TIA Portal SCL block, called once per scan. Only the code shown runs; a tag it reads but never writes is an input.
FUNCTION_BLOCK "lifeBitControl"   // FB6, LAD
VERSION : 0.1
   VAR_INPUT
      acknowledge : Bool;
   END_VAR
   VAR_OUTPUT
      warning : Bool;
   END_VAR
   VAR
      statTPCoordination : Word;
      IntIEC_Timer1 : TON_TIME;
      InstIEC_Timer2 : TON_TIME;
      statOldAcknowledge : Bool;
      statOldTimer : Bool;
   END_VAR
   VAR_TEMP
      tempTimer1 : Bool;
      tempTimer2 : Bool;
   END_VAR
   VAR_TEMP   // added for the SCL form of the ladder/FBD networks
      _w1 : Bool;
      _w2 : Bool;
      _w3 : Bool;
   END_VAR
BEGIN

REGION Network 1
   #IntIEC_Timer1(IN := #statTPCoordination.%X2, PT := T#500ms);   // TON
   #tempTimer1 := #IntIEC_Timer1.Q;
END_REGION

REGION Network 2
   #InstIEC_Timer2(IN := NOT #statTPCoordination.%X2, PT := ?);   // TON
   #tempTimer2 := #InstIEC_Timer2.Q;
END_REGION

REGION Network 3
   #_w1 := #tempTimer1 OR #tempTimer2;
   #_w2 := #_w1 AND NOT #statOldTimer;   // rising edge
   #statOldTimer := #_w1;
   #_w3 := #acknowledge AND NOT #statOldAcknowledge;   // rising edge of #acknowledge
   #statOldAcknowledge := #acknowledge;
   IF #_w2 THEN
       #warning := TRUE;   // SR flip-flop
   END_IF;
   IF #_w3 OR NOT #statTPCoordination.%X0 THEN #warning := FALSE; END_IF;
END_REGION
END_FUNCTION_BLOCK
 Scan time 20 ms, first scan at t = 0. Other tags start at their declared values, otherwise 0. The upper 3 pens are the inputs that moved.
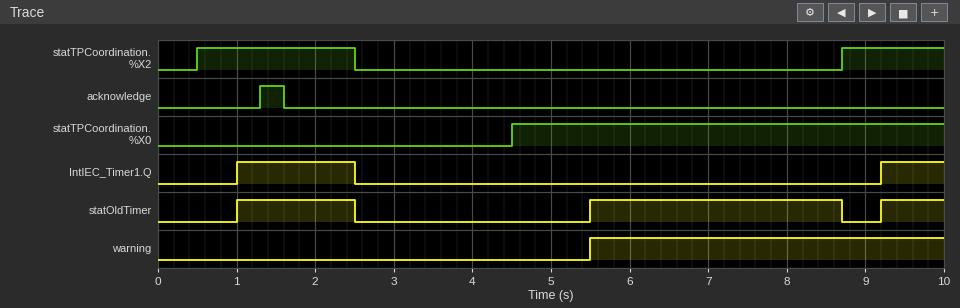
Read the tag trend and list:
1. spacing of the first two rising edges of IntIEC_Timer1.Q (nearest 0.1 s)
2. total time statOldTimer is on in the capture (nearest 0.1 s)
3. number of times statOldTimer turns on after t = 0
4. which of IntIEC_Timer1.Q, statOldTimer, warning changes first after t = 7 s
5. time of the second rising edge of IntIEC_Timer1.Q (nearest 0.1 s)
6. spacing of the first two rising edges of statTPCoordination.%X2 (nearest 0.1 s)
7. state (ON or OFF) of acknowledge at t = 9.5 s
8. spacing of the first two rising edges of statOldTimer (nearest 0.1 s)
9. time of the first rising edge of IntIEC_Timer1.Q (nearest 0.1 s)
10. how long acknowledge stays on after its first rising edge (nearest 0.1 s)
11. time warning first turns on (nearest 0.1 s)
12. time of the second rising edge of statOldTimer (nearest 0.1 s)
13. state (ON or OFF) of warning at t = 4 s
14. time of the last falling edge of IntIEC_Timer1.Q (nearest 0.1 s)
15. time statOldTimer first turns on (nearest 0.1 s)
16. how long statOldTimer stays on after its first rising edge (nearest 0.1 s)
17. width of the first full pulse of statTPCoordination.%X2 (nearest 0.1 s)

8.2 s
5.5 s
3
statOldTimer
9.2 s
8.2 s
OFF
4.5 s
1.0 s
0.3 s
5.5 s
5.5 s
OFF
2.5 s
1.0 s
1.5 s
2.0 s
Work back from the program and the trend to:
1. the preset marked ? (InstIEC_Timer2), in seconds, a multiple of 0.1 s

3.0 s
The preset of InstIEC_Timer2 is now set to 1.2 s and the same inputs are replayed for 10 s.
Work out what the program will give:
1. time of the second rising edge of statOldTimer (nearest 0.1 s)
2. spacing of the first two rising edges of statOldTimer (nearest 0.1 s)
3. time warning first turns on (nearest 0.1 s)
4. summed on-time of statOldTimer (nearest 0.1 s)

3.7 s
2.7 s
9.2 s
7.3 s
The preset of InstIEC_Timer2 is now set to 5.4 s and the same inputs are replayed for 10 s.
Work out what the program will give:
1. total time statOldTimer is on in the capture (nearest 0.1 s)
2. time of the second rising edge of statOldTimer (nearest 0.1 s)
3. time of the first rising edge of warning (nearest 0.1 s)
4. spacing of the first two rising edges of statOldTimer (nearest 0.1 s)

3.1 s
7.9 s
7.9 s
6.9 s
